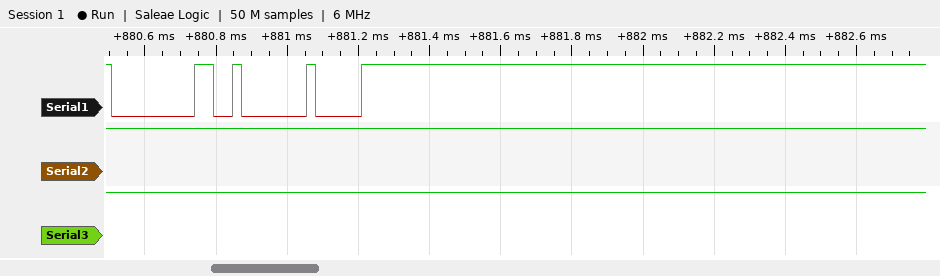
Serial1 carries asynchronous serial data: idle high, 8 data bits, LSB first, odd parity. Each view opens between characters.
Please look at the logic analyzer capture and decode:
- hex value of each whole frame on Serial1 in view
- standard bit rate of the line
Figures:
00, 02, F0
38400 baud
